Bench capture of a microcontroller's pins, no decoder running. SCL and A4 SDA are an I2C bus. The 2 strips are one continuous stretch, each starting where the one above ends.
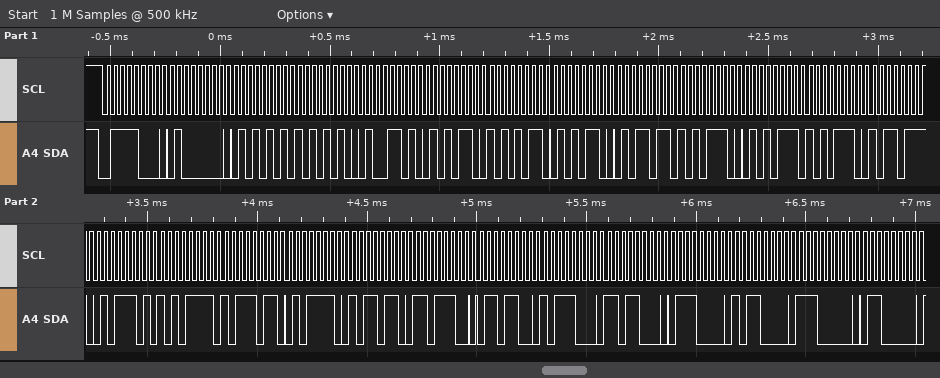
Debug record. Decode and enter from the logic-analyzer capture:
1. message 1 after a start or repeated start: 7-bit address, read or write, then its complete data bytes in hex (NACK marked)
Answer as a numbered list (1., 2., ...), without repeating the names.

1. 0x3C write: 40 55 AA 4D 56 AB 56 5B AE 57 AE B7 5D AF BB 5E B6 DC 6C B8 D8 70 B0 E0 60
